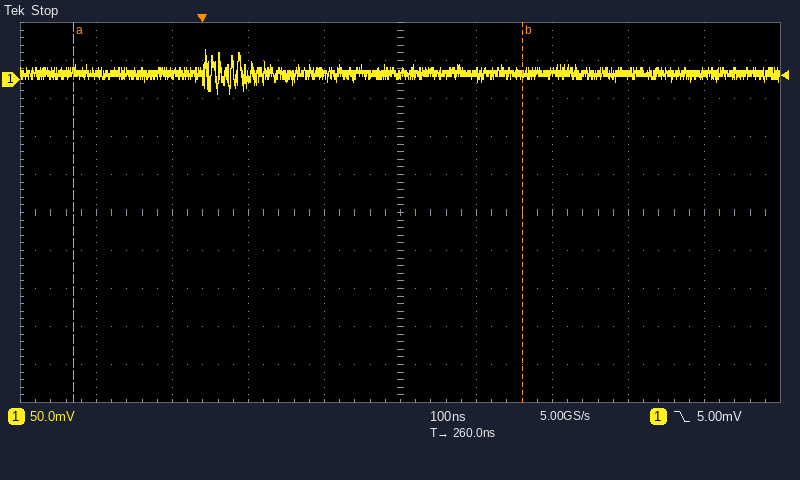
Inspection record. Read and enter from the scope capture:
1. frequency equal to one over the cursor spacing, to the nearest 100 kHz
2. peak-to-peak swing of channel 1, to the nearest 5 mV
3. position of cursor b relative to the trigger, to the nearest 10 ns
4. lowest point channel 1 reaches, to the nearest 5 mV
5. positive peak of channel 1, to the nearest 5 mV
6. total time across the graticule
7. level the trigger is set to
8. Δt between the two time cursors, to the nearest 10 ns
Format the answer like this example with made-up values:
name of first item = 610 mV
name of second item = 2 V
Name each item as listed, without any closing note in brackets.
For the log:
frequency equal to one over the cursor spacing, to the nearest 100 kHz = 1.7 MHz
peak-to-peak swing of channel 1, to the nearest 5 mV = 60 mV
position of cursor b relative to the trigger, to the nearest 10 ns = +420 ns
lowest point channel 1 reaches, to the nearest 5 mV = -20 mV
positive peak of channel 1, to the nearest 5 mV = 40 mV
total time across the graticule = 1 µs
level the trigger is set to = 5.00 mV
Δt between the two time cursors, to the nearest 10 ns = 590 ns
